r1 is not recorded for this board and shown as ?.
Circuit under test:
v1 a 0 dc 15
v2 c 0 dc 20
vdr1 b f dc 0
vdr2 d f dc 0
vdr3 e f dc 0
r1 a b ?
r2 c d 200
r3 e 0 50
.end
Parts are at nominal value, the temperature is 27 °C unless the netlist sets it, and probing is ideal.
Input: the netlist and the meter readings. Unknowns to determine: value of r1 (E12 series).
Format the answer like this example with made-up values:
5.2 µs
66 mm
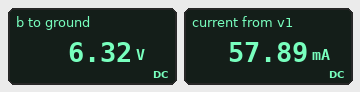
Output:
150 Ω
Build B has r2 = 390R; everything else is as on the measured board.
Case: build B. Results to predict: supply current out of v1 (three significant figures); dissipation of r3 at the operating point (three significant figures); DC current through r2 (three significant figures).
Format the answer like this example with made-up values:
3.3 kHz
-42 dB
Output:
65.5 mA
536 mW
38.0 mA
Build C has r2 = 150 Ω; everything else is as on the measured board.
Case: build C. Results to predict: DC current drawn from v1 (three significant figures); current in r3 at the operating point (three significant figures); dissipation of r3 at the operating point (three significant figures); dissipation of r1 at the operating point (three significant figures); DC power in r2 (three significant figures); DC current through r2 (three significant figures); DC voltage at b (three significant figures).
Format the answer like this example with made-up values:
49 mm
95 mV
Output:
53.3 mA
140 mA
980 mW
427 mW
1.13 W
86.7 mA
7.00 V
